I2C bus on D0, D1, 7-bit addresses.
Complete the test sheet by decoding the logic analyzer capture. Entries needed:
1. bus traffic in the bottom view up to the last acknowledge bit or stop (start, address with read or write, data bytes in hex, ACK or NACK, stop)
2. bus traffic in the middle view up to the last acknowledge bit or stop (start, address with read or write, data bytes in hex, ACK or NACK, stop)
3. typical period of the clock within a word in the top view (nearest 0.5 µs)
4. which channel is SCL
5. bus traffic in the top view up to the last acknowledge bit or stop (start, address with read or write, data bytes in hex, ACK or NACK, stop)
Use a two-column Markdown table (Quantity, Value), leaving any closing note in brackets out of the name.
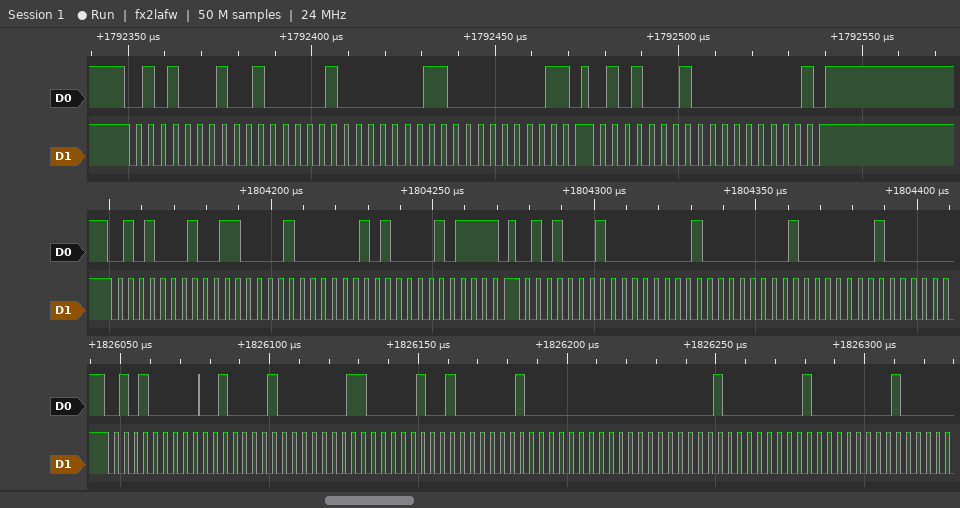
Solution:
| Quantity | Value |
|---|---|
| bus traffic in the bottom view up to the last acknowledge bit or stop | start, address 28 write ACK, 21 ACK, 03 ACK, 09 ACK, 04 ACK, 00 ACK, 01 ACK, 01 ACK, 01 ACK |
| bus traffic in the middle view up to the last acknowledge bit or stop | start, address 28 read ACK, 61 ACK, 05 ACK, 17 NACK, stop, start, address 28 read ACK, 01 ACK, 01 ACK, 02 ACK |
| typical period of the clock within a word in the top view | 3.5 µs |
| which channel is SCL | D1 |
| bus traffic in the top view up to the last acknowledge bit or stop | start, address 28 read ACK, 41 ACK, 03 ACK, 01 NACK, stop, start, address 28 read ACK, 00 NACK, stop |
